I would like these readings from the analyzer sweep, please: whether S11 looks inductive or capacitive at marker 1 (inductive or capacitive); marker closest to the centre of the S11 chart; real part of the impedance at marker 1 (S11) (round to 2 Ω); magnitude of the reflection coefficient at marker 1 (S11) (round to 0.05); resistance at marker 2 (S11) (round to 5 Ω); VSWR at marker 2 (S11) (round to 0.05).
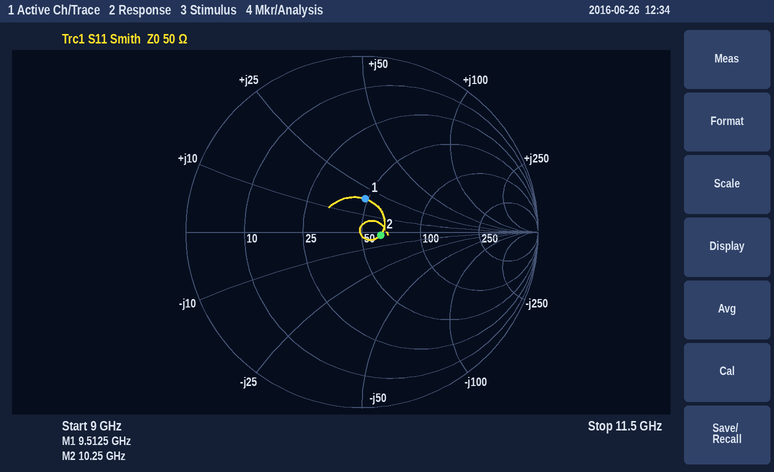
inductive
marker 2
48 Ω
0.20
60 Ω
1.25
